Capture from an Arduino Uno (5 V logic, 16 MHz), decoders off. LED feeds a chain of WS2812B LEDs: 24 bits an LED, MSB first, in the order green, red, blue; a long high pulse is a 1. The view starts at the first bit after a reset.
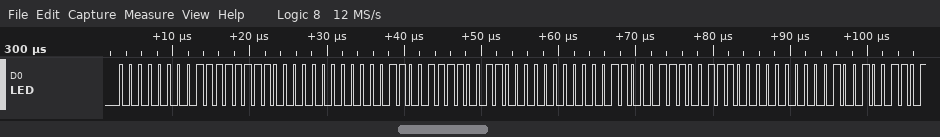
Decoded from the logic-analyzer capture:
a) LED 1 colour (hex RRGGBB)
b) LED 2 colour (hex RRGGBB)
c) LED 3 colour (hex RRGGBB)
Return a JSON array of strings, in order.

["#FF0000", "#F30C00", "#E71800"]
